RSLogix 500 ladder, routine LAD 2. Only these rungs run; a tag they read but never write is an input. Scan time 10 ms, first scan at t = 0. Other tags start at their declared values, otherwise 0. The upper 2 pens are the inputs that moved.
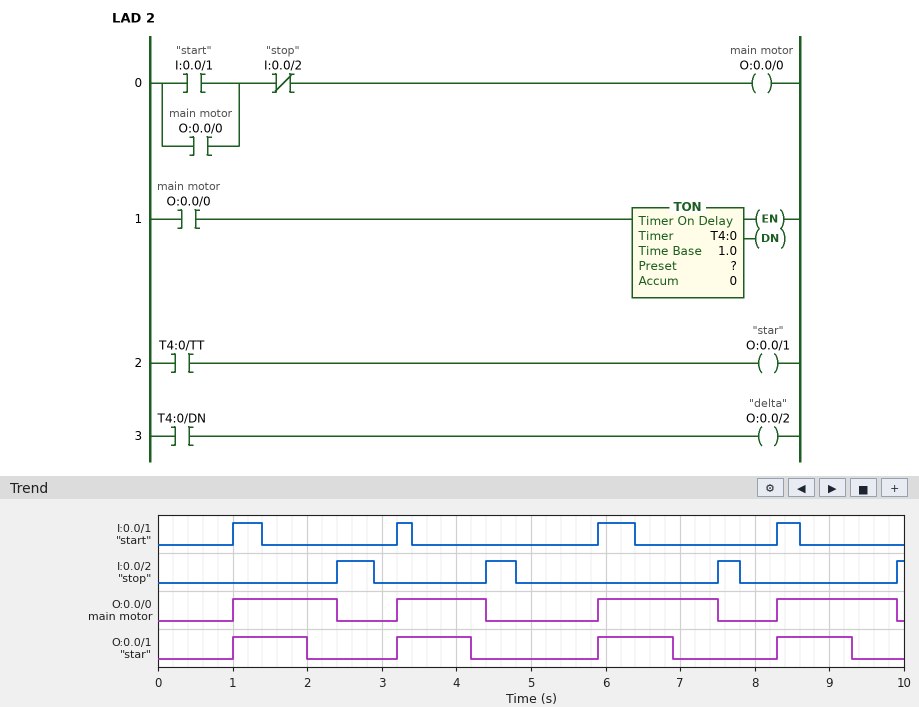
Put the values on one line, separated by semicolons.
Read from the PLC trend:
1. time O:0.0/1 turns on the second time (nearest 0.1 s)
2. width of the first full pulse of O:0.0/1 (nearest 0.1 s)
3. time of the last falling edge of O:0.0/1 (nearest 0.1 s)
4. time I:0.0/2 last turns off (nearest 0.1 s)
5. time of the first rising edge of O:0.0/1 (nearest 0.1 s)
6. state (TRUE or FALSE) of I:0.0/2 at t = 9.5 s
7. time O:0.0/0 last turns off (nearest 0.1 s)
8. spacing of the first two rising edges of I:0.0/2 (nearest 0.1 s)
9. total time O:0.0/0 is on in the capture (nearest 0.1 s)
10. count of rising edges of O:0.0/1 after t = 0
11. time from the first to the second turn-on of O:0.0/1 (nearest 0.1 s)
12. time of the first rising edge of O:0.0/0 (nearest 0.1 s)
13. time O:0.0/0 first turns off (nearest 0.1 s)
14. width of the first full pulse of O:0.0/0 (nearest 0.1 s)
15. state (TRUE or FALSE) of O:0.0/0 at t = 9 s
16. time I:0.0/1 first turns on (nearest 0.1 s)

3.2 s; 1.0 s; 9.3 s; 7.8 s; 1.0 s; FALSE; 9.9 s; 2.0 s; 5.8 s; 4; 2.2 s; 1.0 s; 2.4 s; 1.4 s; TRUE; 1.0 s
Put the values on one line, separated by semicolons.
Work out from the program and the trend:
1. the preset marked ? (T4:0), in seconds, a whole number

1 s
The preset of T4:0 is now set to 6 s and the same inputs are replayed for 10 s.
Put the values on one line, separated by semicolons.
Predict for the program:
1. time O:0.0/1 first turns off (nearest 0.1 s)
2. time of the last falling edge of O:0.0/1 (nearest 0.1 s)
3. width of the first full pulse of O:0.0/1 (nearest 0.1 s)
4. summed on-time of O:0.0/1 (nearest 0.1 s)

2.4 s; 9.9 s; 1.4 s; 5.8 s
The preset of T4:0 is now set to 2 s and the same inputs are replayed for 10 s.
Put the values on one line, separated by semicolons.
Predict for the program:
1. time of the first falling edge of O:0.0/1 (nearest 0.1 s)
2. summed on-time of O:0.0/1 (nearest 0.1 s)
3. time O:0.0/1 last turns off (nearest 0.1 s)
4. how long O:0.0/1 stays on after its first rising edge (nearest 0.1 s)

2.4 s; 5.8 s; 9.9 s; 1.4 s
